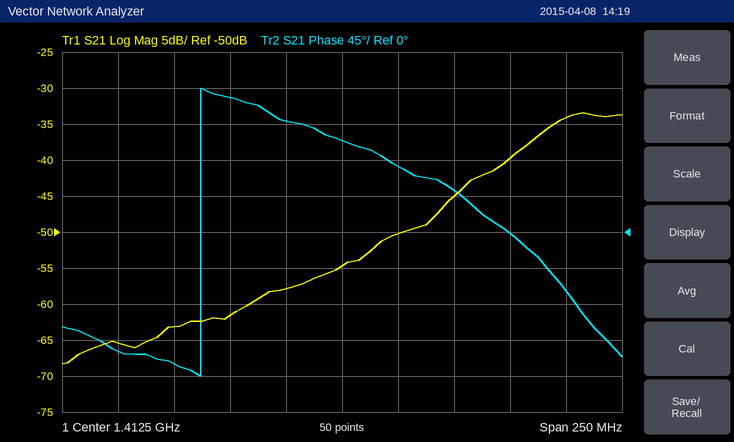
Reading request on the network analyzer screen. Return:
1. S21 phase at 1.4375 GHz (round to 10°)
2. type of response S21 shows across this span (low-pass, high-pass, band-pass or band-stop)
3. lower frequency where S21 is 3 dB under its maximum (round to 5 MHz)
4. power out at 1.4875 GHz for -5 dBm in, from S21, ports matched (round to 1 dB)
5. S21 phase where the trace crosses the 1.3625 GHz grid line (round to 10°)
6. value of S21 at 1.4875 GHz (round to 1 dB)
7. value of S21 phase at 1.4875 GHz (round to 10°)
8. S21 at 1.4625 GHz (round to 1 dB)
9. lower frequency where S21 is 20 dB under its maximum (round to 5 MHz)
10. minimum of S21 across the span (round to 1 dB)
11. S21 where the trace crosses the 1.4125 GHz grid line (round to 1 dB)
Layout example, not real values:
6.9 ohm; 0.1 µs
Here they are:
80°; high-pass; 1.500 GHz; -45 dBm; 170°; -40 dB; 0°; -45 dB; 1.420 GHz; -68 dB; -55 dB
